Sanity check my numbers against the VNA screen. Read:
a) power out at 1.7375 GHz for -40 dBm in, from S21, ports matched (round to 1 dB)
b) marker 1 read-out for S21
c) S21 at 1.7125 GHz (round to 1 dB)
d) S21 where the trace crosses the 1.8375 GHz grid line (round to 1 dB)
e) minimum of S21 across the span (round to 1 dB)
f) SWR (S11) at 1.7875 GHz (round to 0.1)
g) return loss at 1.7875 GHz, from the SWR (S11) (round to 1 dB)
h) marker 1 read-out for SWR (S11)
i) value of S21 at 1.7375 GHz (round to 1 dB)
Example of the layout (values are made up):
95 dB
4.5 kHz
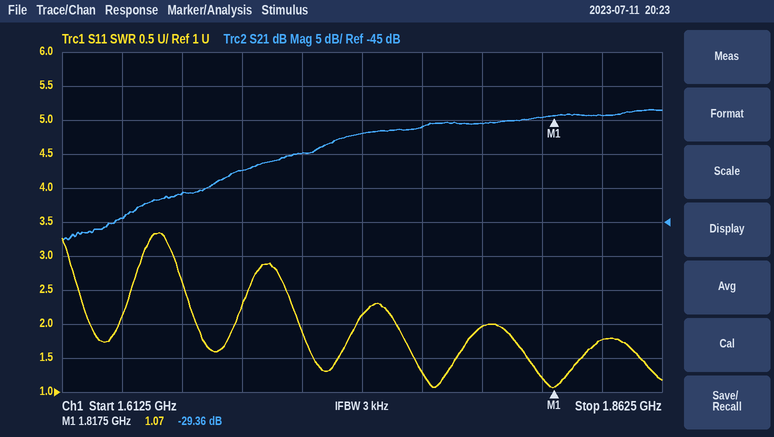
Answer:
-72 dBm
-29.36 dB
-35 dB
-29 dB
-48 dB
2.0
10 dB
1.07
-32 dB
